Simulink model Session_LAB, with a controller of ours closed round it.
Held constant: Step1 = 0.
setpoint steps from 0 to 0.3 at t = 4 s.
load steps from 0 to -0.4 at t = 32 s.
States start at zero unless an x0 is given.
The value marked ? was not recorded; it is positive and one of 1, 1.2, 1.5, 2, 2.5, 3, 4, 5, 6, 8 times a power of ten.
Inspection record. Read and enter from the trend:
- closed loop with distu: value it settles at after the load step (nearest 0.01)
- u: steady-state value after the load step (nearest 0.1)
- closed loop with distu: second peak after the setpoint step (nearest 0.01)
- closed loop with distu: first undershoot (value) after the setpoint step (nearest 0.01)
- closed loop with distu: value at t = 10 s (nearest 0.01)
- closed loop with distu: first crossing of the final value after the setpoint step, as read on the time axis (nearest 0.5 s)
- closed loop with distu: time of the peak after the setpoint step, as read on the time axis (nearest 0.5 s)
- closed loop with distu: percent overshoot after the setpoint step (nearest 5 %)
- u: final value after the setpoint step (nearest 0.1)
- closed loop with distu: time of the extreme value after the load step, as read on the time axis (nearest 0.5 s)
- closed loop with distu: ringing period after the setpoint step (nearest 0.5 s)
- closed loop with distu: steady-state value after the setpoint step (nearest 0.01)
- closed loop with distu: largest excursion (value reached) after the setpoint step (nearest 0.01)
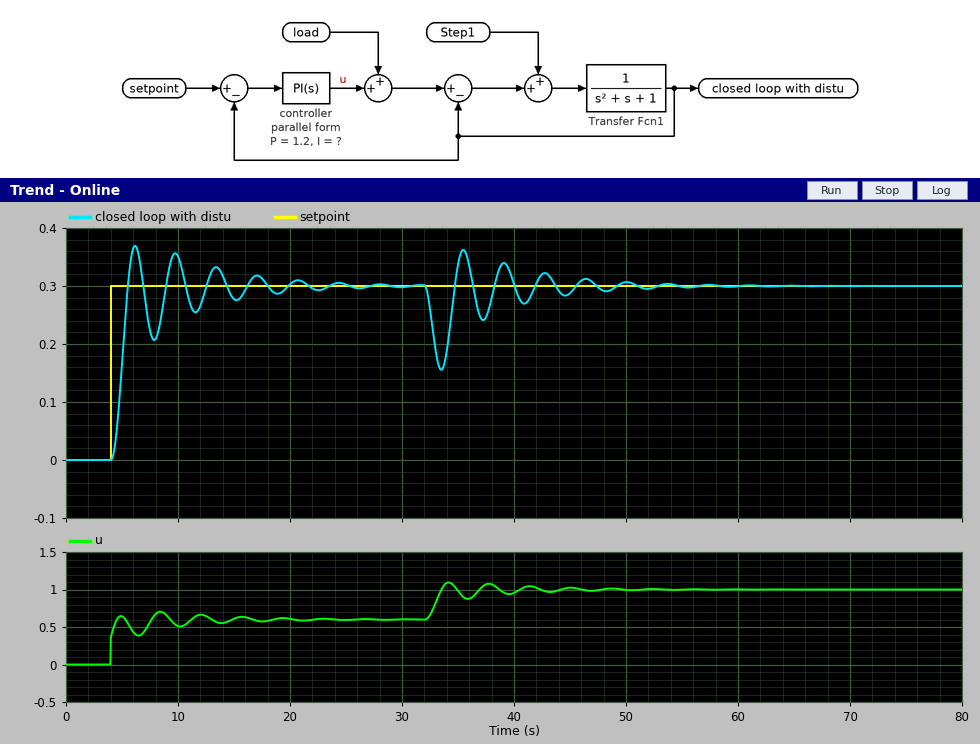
0.30
1.0
0.36
0.21
0.35
5.5 s
6.0 s
25 %
0.6
33.5 s
3.5 s
0.30
0.37
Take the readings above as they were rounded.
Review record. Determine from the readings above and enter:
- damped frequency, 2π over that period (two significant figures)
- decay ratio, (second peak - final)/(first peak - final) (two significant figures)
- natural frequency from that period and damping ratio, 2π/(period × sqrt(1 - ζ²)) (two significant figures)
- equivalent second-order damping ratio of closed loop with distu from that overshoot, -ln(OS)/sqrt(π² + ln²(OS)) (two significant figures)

1.8 rad/s
0.86
2.0 rad/s
0.40
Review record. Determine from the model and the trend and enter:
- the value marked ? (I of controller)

2
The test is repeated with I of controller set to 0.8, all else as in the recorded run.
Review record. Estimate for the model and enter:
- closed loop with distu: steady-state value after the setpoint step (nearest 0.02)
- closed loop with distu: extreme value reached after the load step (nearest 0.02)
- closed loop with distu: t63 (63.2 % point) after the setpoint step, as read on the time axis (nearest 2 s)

0.30
0.14
6 s
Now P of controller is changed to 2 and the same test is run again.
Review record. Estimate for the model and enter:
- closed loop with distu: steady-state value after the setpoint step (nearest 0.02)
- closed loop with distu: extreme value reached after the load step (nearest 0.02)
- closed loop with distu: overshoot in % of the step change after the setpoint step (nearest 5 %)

0.30
0.18
20 %
